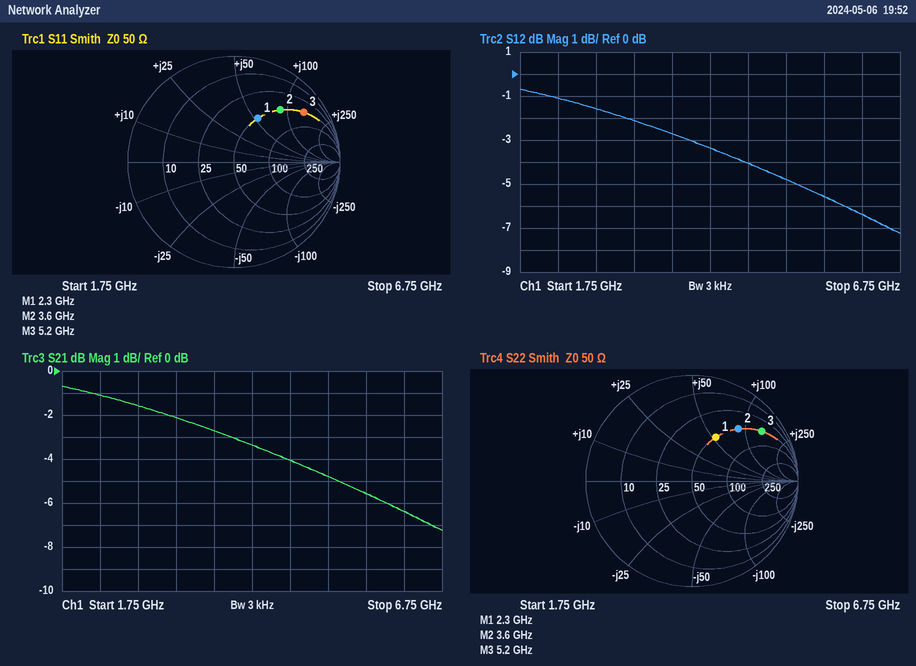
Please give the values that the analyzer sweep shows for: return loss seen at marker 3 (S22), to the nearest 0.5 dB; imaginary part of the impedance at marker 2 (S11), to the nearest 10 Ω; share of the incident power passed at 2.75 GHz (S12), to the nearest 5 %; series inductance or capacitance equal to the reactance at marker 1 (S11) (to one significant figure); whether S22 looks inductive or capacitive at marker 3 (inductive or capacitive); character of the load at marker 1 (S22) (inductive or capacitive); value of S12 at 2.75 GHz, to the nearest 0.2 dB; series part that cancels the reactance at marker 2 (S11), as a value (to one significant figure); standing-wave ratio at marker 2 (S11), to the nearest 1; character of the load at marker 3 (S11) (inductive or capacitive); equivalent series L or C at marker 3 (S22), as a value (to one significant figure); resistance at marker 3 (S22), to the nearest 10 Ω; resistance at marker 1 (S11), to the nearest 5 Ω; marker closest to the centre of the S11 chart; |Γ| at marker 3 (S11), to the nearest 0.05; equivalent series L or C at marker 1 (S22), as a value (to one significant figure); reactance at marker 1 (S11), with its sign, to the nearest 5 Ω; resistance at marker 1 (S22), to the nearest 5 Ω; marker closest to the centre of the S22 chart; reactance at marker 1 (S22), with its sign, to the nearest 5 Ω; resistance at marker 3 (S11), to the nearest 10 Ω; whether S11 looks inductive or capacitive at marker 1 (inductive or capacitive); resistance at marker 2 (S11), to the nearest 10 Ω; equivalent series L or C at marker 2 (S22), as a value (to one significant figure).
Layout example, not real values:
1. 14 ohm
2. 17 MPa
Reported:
1. 2.0 dB
2. +90 Ω
3. 70 %
4. 4 nH
5. inductive
6. inductive
7. -1.6 dB
8. 500 fF
9. 5
10. inductive
11. 4 nH
12. 50 Ω
13. 50 Ω
14. marker 1
15. 0.80
16. 4 nH
17. +55 Ω
18. 50 Ω
19. marker 1
20. +55 Ω
21. 50 Ω
22. inductive
23. 50 Ω
24. 4 nH
